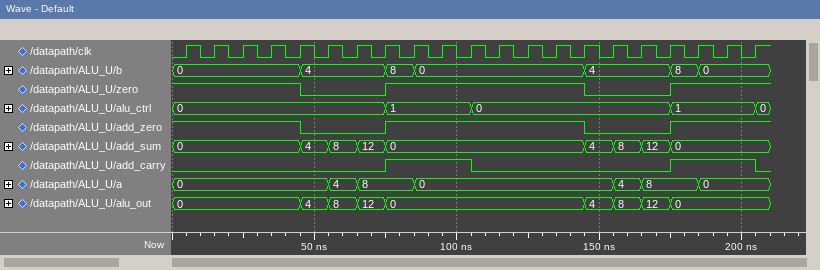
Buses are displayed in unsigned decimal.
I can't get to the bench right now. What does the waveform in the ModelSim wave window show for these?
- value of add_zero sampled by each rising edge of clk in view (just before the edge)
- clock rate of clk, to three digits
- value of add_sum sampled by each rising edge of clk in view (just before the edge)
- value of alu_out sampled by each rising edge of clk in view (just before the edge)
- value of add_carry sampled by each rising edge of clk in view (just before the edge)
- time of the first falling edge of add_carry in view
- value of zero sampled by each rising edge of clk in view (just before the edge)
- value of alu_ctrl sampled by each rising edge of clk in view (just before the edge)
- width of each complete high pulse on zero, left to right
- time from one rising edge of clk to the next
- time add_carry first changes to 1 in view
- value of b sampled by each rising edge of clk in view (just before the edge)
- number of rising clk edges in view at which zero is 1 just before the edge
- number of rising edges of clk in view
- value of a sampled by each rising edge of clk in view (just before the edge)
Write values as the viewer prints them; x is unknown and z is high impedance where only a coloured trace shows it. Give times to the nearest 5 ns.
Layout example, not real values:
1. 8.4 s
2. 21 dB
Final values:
1. 1 1 1 1 1 0 0 0 1 1 1 1 1 1 1 0 0 0 1 1 1
2. 100 MHz
3. 0, 0, 0, 0, 0, 4, 8, 12, 0, 0, 0, 0, 0, 0, 0, 4, 8, 12, 0, 0, 0
4. 0, 0, 0, 0, 0, 4, 8, 12, 0, 0, 0, 0, 0, 0, 0, 4, 8, 12, 0, 0, 0
5. 0 0 0 0 0 0 0 0 1 1 1 0 0 0 0 0 0 0 1 1 1
6. 105 ns
7. 1 1 1 1 1 0 0 0 1 1 1 1 1 1 1 0 0 0 1 1 1
8. 0, 0, 0, 0, 0, 0, 0, 0, 1, 1, 1, 0, 0, 0, 0, 0, 0, 0, 1, 1, 1
9. 70 ns
10. 10 ns
11. 75 ns
12. 0, 0, 0, 0, 0, 4, 4, 4, 8, 0, 0, 0, 0, 0, 0, 4, 4, 4, 8, 0, 0
13. 15
14. 21
15. 0, 0, 0, 0, 0, 0, 4, 8, 8, 0, 0, 0, 0, 0, 0, 0, 4, 8, 8, 0, 0
